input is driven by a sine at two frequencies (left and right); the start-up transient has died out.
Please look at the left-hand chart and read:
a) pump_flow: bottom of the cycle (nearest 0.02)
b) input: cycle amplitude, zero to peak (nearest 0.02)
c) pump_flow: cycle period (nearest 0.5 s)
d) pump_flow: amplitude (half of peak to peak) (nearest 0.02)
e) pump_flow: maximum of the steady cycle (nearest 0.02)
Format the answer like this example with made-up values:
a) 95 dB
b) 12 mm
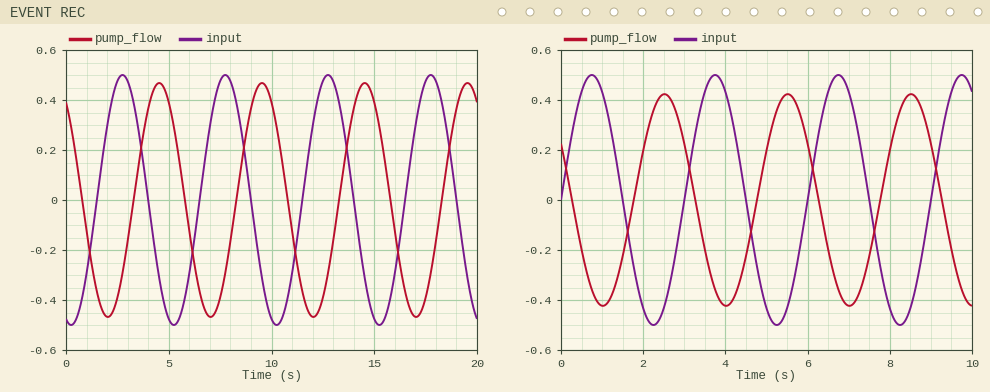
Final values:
a) -0.46
b) 0.50
c) 5.0 s
d) 0.46
e) 0.46
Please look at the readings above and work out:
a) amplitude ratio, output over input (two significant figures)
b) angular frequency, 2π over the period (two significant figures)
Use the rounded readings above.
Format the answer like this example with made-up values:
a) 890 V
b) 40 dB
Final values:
a) 0.92
b) 1.3 rad/s
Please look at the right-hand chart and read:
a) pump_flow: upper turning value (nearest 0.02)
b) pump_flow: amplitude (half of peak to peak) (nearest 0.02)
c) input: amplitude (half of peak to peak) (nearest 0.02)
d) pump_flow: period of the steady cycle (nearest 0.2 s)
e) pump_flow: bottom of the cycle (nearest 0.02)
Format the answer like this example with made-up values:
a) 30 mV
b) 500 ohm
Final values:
a) 0.42
b) 0.42
c) 0.50
d) 3.0 s
e) -0.42
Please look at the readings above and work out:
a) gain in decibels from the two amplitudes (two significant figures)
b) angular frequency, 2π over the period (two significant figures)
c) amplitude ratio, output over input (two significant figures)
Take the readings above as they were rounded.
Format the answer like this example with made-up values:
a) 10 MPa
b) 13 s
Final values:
a) -1.5 dB
b) 2.1 rad/s
c) 0.84
